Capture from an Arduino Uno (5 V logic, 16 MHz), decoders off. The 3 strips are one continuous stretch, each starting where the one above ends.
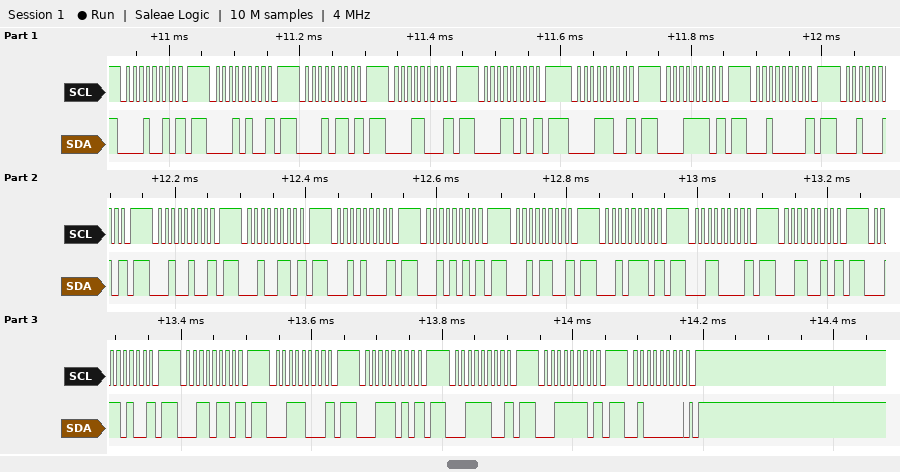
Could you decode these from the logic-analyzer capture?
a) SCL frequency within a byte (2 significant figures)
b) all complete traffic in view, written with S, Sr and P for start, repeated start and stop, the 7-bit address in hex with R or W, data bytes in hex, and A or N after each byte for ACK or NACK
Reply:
100 kHz
S 09W N P S 0AW N P S 0BW N P S 0CW N P S 0DW N P S 0EW N P S 0FW N P S 10W N P S 11W N P S 12W N P S 13W N P S 14W N P S 15W N P S 16W N P S 17W N P S 18W N P S 19W N P S 1AW N P S 1BW N P S 1CW N P S 1DW N P S 1EW N P S 1FW N P S 20W A P
